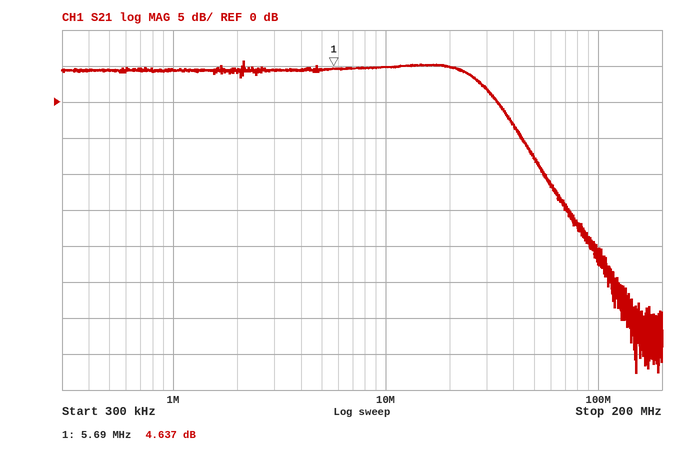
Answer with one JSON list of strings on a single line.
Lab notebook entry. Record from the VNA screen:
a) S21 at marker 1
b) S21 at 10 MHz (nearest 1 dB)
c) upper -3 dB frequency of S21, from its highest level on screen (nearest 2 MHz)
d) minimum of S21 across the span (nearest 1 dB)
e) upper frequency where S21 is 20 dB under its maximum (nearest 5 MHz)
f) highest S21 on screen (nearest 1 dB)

["4.637 dB", "5 dB", "28 MHz", "-38 dB", "70 MHz", "6 dB"]
